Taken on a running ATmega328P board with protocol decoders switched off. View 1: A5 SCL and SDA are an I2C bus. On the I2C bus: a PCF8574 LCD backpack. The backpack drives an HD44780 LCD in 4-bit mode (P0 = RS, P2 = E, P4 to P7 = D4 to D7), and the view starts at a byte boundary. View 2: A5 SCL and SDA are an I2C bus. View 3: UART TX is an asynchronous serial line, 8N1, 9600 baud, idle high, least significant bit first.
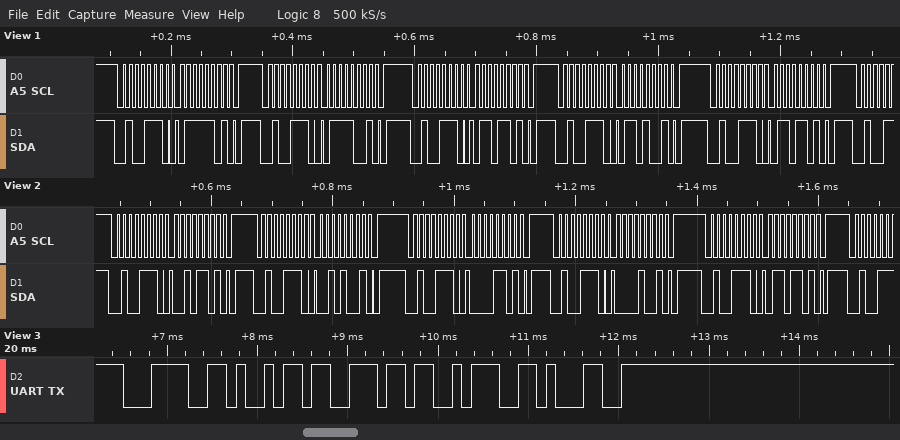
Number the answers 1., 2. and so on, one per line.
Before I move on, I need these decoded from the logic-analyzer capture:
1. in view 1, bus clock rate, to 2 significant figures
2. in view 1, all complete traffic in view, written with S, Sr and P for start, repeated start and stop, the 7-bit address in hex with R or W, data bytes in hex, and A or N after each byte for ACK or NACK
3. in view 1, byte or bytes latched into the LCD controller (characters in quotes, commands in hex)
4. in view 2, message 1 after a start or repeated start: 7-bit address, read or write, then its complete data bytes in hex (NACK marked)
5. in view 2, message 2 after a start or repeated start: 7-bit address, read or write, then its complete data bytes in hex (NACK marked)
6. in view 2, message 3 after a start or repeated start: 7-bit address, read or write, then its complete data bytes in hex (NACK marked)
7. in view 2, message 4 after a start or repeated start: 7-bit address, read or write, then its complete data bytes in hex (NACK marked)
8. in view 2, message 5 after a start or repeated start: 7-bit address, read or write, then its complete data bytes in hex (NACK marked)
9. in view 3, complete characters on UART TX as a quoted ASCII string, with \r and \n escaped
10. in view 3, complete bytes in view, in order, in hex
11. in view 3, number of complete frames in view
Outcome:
1. 100 kHz
2. S 27W A 7D A P S 27W A 79 A P S 27W A 6D A P S 27W A 69 A P S 27W A 6D A P
3. 'v'
4. 0x27 write: 2D
5. 0x27 write: 29
6. 0x27 write: 0D
7. 0x27 write: 09
8. 0x27 write: 6D
9. "<in:1"
10. 3C 69 6E 3A 31
11. 5
